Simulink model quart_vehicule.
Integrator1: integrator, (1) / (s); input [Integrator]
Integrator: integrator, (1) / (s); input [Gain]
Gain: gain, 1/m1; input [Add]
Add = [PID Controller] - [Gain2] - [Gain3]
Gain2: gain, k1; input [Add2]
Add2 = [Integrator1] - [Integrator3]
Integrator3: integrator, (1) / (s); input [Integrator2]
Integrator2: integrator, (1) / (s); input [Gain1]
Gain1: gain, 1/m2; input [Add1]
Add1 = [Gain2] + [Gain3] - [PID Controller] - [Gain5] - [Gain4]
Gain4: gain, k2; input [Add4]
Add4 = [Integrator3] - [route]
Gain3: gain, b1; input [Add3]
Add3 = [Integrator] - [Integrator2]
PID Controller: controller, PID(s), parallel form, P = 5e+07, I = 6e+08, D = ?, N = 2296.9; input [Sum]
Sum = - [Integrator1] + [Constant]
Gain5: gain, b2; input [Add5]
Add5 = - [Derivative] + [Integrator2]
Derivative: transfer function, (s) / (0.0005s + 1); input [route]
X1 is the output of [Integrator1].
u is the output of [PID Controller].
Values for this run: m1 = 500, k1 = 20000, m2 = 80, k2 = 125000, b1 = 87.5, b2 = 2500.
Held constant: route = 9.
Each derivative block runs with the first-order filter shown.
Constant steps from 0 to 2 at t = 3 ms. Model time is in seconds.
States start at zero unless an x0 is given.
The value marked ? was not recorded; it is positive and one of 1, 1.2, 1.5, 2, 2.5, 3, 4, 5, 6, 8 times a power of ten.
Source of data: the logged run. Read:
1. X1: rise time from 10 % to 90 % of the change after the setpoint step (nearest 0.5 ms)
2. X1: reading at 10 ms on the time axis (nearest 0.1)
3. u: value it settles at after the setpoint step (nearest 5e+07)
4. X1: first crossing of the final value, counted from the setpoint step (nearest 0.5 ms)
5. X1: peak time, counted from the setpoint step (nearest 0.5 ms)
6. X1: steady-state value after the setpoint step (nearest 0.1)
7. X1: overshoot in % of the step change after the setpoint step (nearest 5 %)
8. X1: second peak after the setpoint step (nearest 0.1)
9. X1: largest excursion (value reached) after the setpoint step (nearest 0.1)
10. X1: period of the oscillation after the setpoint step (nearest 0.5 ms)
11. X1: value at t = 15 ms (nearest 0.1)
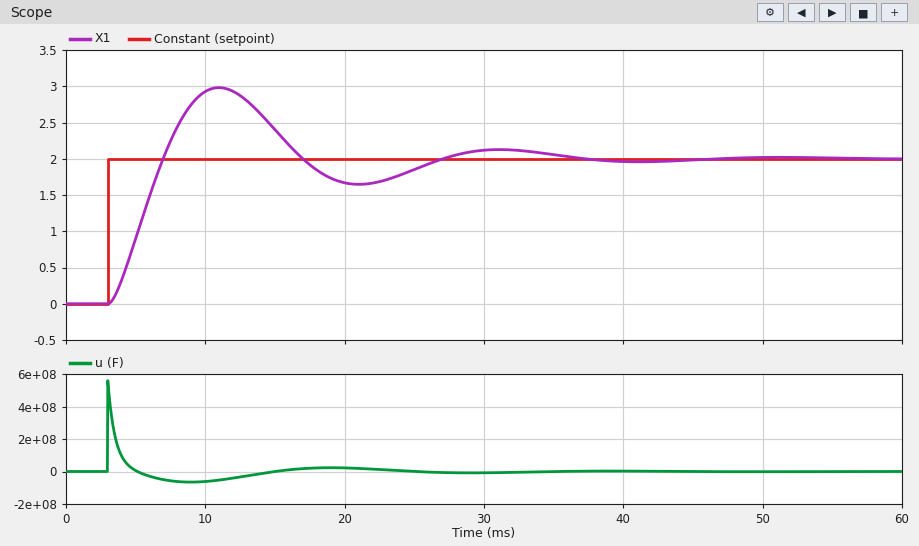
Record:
3.0 ms
2.9
0
4.0 ms
8.0 ms
2.0
50 %
2.1
3.0
20.0 ms
2.4
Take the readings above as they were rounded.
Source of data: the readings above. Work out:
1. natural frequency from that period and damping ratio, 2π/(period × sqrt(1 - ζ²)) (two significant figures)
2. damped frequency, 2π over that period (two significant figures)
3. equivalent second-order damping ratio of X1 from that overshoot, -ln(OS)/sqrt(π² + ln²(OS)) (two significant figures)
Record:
0.32 rad/ms
0.31 rad/ms
0.22
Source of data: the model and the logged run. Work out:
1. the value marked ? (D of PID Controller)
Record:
100000
